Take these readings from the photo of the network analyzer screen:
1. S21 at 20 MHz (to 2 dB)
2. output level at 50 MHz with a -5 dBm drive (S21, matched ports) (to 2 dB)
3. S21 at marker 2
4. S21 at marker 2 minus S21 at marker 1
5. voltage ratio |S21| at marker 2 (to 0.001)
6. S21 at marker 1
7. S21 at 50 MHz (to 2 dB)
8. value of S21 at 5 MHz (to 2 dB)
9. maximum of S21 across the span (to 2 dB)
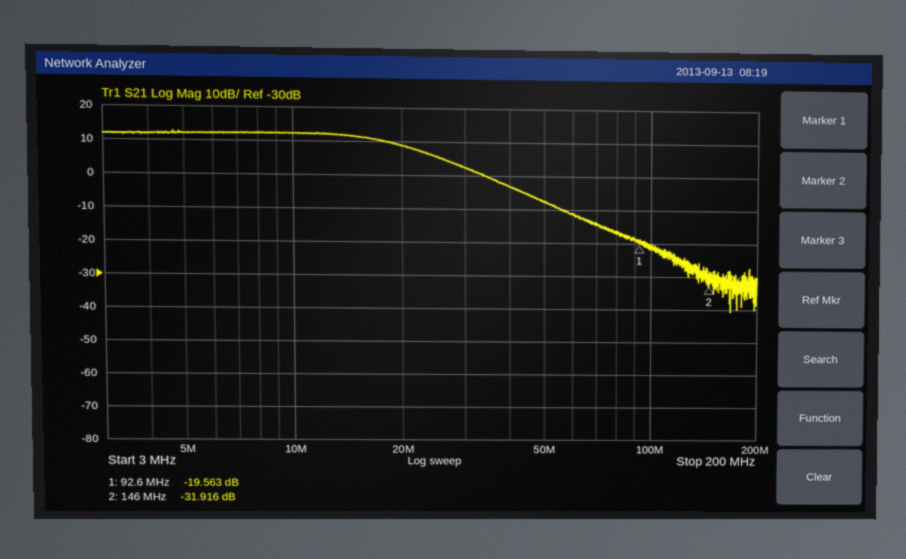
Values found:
8 dB
-12 dBm
-31.916 dB
-12.353 dB
0.025
-19.563 dB
-8 dB
12 dB
12 dB
